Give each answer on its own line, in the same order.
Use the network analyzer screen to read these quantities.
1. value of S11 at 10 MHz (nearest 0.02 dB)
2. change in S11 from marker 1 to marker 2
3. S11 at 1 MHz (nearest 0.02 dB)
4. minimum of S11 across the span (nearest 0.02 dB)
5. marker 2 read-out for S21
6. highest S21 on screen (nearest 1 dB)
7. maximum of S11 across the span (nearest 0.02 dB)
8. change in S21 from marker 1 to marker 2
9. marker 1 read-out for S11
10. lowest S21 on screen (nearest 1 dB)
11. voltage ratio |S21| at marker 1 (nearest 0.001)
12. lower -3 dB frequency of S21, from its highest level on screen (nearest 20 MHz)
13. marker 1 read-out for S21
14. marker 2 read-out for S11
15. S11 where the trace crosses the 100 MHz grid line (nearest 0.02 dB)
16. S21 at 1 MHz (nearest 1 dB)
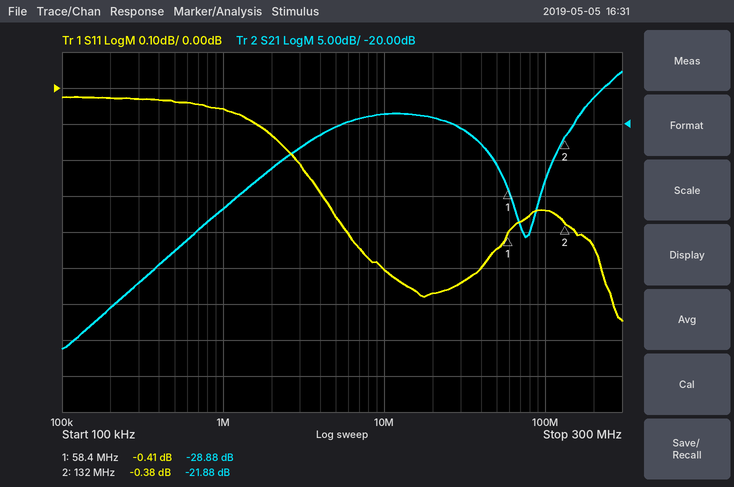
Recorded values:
-0.50 dB
0.03 dB
-0.06 dB
-0.64 dB
-21.88 dB
-13 dB
-0.02 dB
7.00 dB
-0.41 dB
-51 dB
0.036
220 MHz
-28.88 dB
-0.38 dB
-0.34 dB
-32 dB
